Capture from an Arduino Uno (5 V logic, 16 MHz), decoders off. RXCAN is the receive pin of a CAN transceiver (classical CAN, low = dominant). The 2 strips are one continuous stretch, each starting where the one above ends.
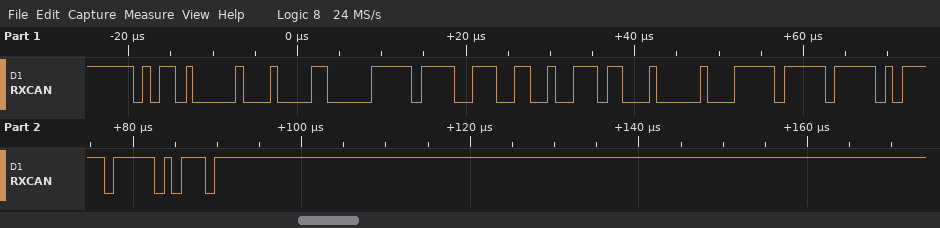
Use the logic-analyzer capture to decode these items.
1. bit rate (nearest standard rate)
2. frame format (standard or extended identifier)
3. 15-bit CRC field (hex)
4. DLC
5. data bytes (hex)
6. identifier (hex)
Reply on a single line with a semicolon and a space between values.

1000 kbit/s; standard; 0x3FFB; 8; 60 FF 39 93 B1 00 FF FF; 0x5A0
